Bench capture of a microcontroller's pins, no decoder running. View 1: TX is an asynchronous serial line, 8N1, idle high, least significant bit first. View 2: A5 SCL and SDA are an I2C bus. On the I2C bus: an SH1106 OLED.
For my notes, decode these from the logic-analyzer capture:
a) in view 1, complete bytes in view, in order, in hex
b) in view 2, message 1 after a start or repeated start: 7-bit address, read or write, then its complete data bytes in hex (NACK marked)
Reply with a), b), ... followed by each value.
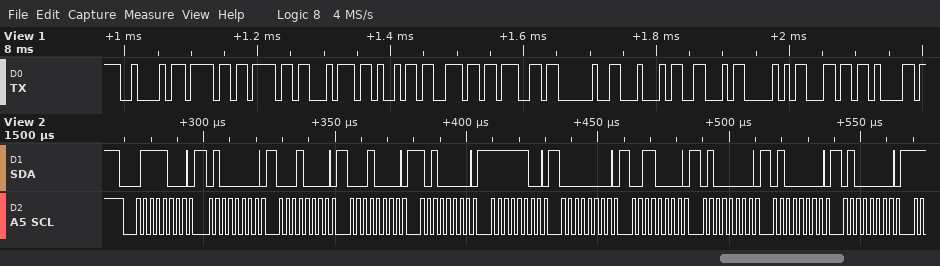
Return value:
a) 42 6F 6F 74 69 6E 67 20 44 46 50 6C 61
b) 0x3C write: 40 10 10 A0 FC 00 30 40 40 40
